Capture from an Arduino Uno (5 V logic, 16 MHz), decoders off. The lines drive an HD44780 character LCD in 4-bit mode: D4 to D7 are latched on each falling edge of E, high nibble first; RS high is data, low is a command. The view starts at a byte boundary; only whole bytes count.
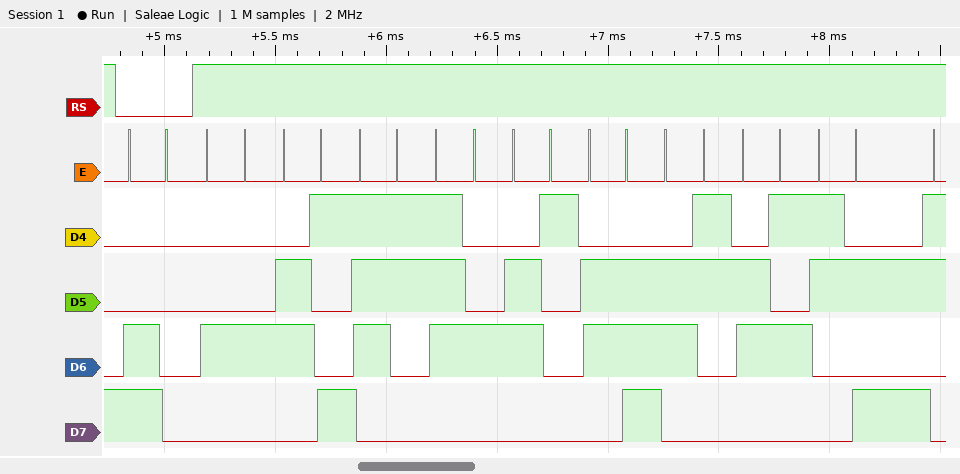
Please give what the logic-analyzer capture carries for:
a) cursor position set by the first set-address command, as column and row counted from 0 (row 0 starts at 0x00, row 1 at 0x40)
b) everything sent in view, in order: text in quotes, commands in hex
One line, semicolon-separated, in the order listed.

column 0, row 1; 0xC0 "Distance:"
